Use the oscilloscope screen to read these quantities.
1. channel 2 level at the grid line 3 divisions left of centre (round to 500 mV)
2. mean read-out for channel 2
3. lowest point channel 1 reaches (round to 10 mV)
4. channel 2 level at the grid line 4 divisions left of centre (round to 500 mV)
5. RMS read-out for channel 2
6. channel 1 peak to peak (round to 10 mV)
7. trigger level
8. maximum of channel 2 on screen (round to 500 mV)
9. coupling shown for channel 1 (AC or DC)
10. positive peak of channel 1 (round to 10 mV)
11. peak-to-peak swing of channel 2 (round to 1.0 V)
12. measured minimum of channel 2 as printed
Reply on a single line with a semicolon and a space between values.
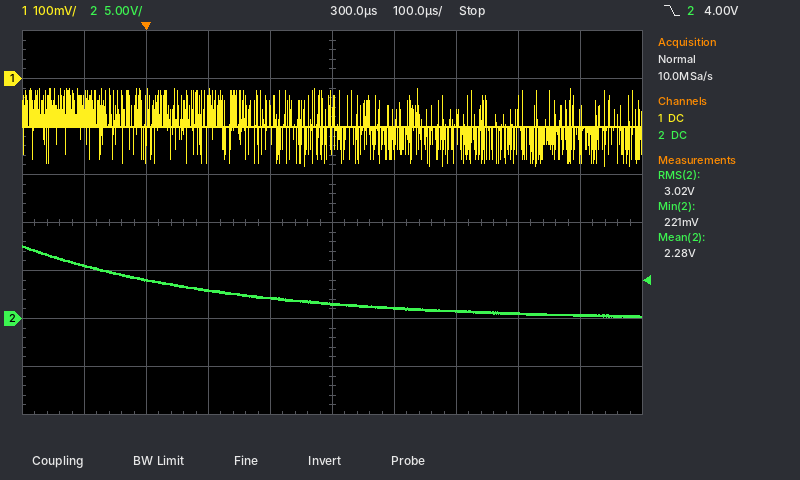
4.0 V; 2.28 V; -180 mV; 5.5 V; 3.02 V; 160 mV; 4.00 V; 7.5 V; DC; -20 mV; 7.0 V; 221 mV
